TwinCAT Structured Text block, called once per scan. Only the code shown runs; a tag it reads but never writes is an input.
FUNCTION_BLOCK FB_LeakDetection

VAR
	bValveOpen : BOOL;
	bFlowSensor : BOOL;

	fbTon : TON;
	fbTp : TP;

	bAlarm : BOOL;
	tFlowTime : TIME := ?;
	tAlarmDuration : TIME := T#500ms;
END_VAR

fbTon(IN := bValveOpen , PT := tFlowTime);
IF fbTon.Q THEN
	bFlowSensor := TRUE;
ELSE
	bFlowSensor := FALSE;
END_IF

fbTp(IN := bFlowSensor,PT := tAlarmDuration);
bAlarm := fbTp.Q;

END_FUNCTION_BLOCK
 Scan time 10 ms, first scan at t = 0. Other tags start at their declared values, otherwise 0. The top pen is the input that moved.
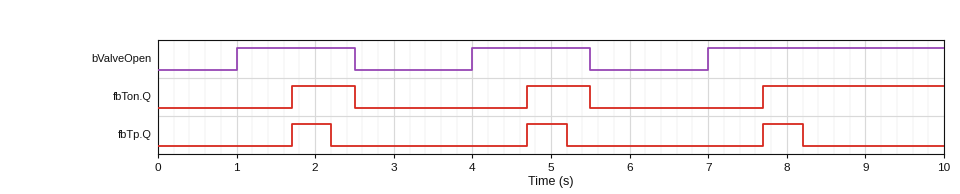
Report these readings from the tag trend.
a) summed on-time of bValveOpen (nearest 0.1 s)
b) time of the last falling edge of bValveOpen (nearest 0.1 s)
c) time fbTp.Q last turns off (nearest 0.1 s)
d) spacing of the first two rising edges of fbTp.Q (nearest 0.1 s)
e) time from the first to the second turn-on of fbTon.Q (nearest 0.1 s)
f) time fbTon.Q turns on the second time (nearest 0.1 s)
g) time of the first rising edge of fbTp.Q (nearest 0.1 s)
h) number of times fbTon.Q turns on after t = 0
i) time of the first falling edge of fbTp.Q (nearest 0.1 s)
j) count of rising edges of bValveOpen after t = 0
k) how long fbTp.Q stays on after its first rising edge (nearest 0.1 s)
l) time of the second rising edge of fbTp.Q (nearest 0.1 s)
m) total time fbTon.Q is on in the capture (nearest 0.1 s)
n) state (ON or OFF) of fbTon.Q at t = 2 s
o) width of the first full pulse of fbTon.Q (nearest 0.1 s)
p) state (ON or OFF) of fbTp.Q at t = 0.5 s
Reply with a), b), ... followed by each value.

a) 6.0 s
b) 5.5 s
c) 8.2 s
d) 3.0 s
e) 3.0 s
f) 4.7 s
g) 1.7 s
h) 3
i) 2.2 s
j) 3
k) 0.5 s
l) 4.7 s
m) 3.9 s
n) ON
o) 0.8 s
p) OFF
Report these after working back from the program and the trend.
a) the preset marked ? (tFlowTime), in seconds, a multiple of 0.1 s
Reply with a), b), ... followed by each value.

a) 0.7 s
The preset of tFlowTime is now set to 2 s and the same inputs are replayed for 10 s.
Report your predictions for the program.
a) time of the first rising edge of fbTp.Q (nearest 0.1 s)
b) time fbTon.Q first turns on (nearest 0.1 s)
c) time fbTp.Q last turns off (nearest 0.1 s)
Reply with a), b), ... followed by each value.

a) 9.0 s
b) 9.0 s
c) 9.5 s
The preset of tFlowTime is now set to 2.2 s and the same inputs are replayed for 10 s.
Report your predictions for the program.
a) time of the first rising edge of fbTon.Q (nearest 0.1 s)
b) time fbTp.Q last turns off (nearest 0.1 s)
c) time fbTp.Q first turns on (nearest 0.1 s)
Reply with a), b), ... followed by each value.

a) 9.2 s
b) 9.7 s
c) 9.2 s
